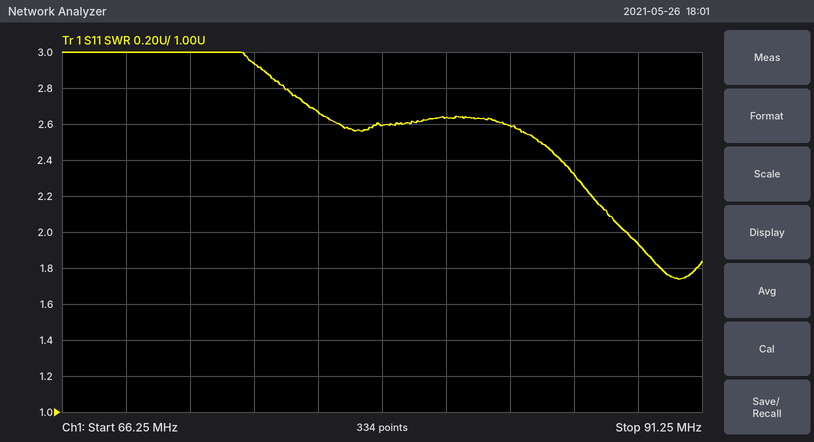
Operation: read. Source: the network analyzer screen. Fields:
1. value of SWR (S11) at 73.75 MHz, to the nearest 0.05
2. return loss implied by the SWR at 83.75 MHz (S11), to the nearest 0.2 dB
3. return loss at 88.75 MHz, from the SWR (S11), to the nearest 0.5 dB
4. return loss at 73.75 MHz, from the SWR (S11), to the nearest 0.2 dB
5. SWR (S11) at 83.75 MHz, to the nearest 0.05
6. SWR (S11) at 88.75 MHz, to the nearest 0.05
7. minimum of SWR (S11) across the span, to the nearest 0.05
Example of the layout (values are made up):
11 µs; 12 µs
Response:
2.95; 7.0 dB; 10.0 dB; 6.2 dB; 2.60; 1.95; 1.75
